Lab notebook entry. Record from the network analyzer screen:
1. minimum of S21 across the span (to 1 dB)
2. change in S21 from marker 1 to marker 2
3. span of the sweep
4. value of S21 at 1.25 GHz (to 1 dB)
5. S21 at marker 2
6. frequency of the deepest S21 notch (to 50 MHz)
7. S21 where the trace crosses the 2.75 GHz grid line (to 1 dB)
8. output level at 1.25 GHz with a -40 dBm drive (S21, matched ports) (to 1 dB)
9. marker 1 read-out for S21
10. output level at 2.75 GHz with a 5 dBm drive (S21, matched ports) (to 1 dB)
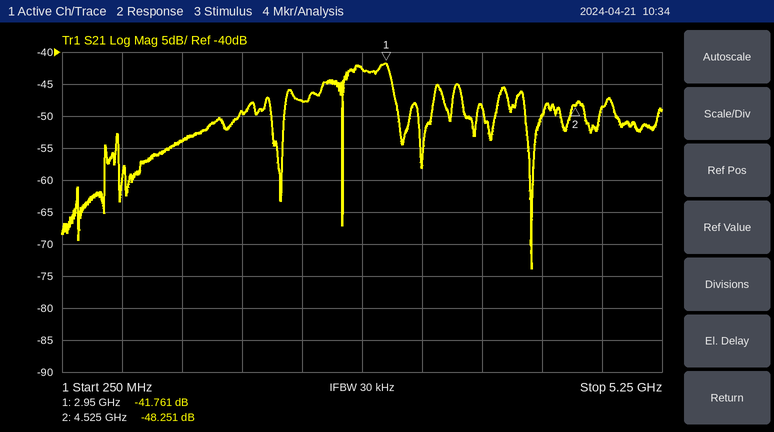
-74 dB
-6.490 dB
5 GHz
-54 dB
-48.251 dB
4.15 GHz
-43 dB
-94 dBm
-41.761 dB
-38 dBm
